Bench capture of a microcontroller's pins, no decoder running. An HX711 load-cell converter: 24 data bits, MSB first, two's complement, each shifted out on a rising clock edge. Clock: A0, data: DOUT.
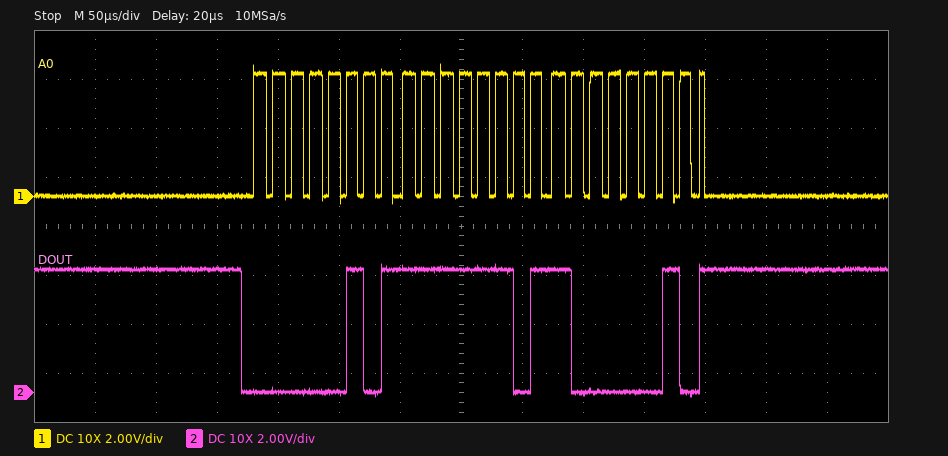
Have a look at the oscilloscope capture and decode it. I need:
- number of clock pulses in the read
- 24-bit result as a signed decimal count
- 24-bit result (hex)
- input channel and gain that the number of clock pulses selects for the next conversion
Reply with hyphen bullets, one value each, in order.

- 25
- 392578
- 0x05FD82
- channel A, gain 128
